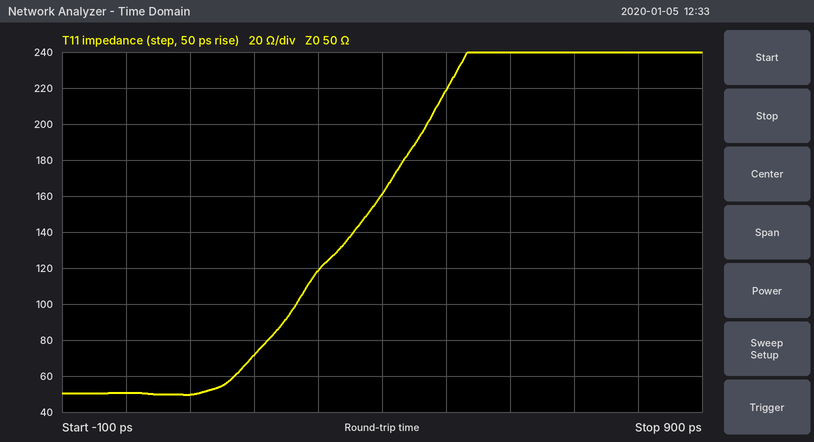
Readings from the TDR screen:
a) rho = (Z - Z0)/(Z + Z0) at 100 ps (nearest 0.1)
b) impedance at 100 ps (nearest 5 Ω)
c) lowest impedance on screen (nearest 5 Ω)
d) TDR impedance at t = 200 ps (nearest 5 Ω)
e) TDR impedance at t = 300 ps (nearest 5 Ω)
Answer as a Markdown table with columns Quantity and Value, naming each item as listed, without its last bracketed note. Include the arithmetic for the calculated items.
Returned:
| Quantity | Value |
|---|---|
| rho = (Z - Z0)/(Z + Z0) at 100 ps | (50 − 50)/(50 + 50) ≈ 0.0 |
| impedance at 100 ps | 50 Ω |
| lowest impedance on screen | 50 Ω |
| TDR impedance at t = 200 ps | 70 Ω |
| TDR impedance at t = 300 ps | 120 Ω |
